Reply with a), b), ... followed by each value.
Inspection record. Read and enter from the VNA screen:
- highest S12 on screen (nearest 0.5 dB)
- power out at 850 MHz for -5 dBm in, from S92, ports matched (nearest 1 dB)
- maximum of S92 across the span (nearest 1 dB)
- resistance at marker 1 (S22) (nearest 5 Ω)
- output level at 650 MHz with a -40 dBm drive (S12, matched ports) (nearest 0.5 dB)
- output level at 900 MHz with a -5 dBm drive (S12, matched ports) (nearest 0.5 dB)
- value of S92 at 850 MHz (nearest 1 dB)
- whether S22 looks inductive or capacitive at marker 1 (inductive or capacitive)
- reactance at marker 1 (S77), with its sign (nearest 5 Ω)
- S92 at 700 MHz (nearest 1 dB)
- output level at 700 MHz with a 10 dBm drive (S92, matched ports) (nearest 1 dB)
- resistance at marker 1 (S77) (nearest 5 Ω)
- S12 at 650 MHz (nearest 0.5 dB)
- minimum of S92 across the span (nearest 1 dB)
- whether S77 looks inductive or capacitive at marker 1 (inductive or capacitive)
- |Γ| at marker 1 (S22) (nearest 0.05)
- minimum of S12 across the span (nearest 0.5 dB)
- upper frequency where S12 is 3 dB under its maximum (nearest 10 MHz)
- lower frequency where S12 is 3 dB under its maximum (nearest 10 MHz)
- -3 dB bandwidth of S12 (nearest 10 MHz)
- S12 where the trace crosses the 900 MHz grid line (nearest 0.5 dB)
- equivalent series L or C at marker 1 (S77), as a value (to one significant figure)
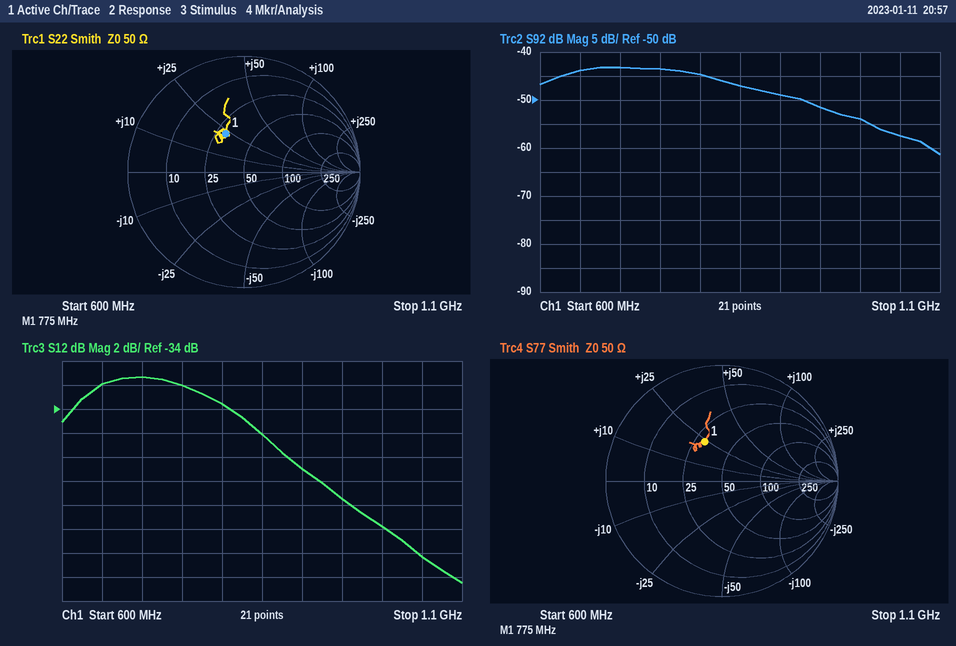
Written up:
a) -31.5 dB
b) -52 dBm
c) -43 dB
d) 30 Ω
e) -72.0 dBm
f) -44.0 dBm
g) -47 dB
h) inductive
i) +25 Ω
j) -43 dB
k) -33 dBm
l) 30 Ω
m) -32.0 dB
n) -61 dB
o) inductive
p) 0.35
q) -48.5 dB
r) 820 MHz
s) 610 MHz
t) 210 MHz
u) -39.0 dB
v) 5 nH
